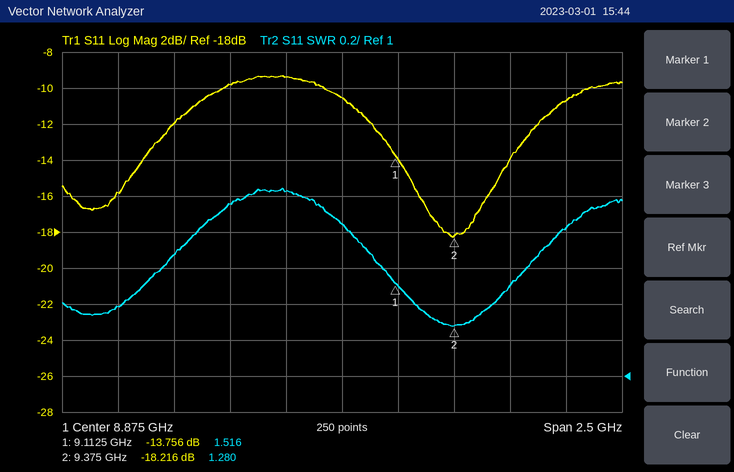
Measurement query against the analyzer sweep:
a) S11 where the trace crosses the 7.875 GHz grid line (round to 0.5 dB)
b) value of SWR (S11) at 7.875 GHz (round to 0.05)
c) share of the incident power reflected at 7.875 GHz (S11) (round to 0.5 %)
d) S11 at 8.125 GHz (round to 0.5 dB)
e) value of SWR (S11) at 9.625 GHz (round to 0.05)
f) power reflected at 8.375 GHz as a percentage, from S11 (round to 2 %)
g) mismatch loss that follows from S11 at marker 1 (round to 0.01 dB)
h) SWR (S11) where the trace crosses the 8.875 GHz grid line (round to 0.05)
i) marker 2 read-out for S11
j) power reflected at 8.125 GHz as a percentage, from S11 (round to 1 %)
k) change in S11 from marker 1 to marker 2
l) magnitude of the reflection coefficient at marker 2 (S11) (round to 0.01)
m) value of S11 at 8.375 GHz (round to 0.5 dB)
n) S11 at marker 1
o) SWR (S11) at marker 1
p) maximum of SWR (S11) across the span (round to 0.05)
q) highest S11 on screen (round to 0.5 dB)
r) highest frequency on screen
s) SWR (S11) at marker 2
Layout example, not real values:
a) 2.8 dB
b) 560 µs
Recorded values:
a) -16.0 dB
b) 1.40
c) 2.5 %
d) -12.0 dB
e) 1.50
f) 10 %
g) 0.19 dB
h) 1.85
i) -18.216 dB
j) 6 %
k) -4.460 dB
l) 0.12
m) -10.0 dB
n) -13.756 dB
o) 1.516
p) 2.05
q) -9.5 dB
r) 10.125 GHz
s) 1.280
